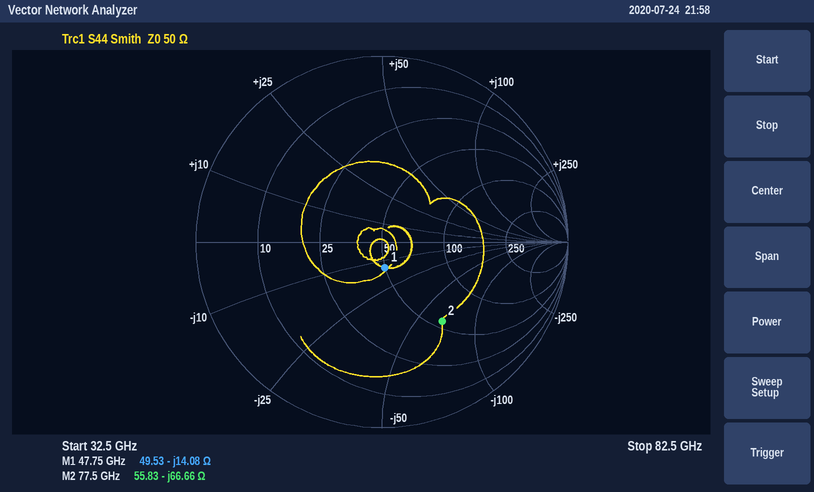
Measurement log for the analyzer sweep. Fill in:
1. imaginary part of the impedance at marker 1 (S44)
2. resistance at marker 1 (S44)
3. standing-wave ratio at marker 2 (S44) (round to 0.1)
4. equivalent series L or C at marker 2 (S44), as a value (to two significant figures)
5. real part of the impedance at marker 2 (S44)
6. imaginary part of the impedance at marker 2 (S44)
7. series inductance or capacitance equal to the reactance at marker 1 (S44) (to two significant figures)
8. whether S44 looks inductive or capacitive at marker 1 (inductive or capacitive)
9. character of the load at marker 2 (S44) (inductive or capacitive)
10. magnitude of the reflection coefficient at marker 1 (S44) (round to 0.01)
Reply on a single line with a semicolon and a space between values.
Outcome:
-14.08 Ω; 49.53 Ω; 3.3; 31 fF; 55.83 Ω; -66.66 Ω; 240 fF; capacitive; capacitive; 0.14
